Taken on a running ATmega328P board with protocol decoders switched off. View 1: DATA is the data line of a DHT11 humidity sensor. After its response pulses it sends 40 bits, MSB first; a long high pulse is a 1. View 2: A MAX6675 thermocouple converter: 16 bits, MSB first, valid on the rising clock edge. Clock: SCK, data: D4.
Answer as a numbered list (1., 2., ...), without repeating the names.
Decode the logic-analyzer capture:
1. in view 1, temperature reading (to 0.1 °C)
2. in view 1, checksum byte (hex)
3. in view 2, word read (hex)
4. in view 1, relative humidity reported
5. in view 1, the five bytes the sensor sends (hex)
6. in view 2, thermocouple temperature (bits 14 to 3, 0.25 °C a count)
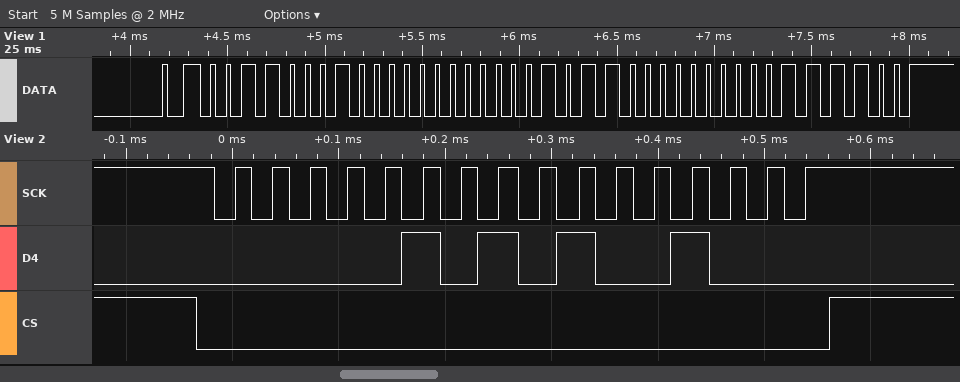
1. 11.0 °C
2. 0x3C
3. 0x0548
4. 49 %
5. 31 00 0B 00 3C
6. 42.25 °C
